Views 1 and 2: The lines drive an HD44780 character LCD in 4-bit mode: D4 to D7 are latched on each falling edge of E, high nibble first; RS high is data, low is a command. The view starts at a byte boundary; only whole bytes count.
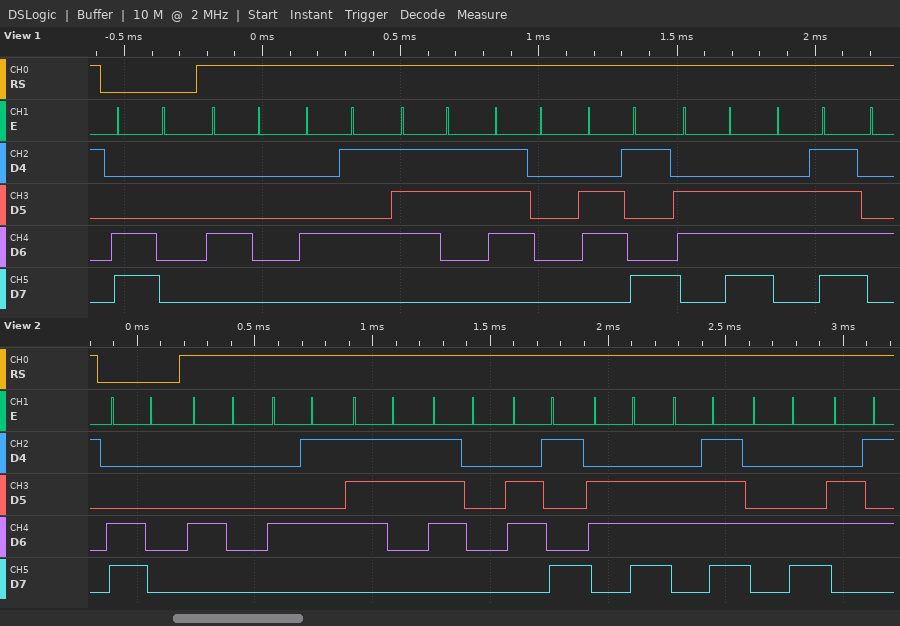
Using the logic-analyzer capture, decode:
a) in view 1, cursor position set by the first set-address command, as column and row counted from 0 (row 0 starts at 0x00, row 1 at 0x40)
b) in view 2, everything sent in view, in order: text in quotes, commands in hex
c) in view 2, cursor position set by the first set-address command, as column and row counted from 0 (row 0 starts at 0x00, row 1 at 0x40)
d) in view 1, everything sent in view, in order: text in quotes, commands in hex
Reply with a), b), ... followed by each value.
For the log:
a) column 0, row 1
b) 0xC0 "@EspinoLe"
c) column 0, row 1
d) 0xC0 "@Espino"
